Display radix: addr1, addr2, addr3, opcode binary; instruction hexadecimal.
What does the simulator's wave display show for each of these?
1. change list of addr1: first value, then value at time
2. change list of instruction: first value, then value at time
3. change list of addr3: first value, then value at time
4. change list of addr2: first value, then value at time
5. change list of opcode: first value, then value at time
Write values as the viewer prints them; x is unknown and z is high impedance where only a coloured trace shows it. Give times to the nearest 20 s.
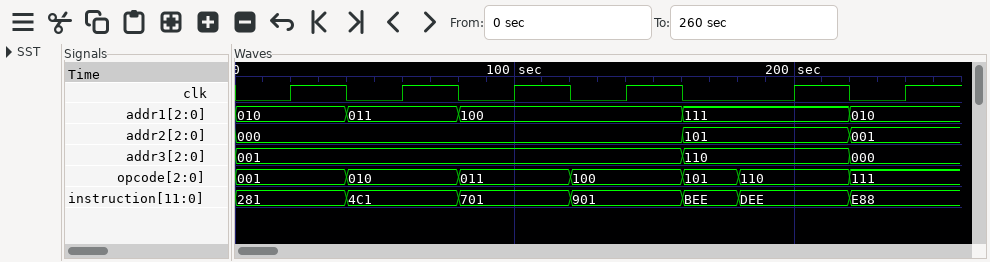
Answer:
010, 011 at 40 s, 100 at 80 s, 111 at 160 s, 010 at 220 s
281, 4C1 at 40 s, 701 at 80 s, 901 at 120 s, BEE at 160 s, DEE at 180 s, E88 at 220 s
001, 110 at 160 s, 000 at 220 s
000, 101 at 160 s, 001 at 220 s
001, 010 at 40 s, 011 at 80 s, 100 at 120 s, 101 at 160 s, 110 at 180 s, 111 at 220 s
